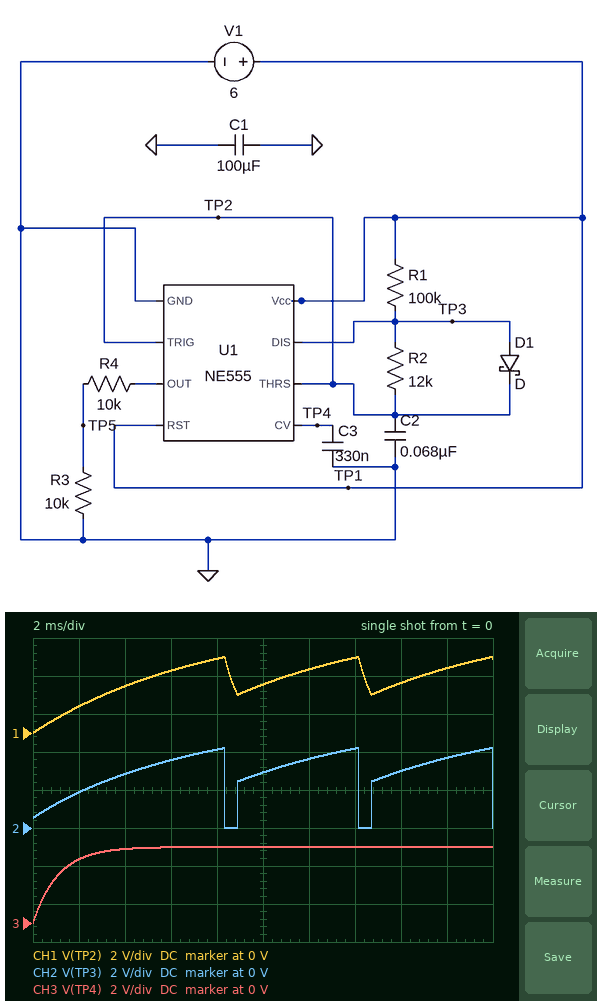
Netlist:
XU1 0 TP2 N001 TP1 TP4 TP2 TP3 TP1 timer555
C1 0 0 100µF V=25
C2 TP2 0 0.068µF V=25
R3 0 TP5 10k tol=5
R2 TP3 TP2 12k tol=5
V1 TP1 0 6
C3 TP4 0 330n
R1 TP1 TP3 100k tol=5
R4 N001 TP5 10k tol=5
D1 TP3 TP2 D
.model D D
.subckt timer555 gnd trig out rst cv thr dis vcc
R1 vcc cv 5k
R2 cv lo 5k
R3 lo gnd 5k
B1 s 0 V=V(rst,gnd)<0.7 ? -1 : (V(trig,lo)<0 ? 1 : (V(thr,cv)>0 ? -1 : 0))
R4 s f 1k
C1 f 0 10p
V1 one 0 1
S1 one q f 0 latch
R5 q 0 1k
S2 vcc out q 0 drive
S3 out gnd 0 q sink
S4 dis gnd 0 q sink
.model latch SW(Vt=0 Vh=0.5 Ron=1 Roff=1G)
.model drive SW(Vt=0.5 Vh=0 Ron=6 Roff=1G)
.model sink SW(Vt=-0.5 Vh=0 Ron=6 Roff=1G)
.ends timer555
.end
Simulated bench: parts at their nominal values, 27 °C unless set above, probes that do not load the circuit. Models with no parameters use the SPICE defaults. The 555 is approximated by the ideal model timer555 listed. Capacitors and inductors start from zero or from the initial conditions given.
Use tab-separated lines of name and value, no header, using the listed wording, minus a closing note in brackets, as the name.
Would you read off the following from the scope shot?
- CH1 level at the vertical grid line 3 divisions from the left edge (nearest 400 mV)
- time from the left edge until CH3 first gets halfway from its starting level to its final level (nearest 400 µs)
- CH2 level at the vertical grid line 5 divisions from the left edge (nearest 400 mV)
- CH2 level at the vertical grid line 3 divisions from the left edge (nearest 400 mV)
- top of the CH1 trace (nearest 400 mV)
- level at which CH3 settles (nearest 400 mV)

CH1 level at the vertical grid line 3 divisions from the left edge	3.2 V
time from the left edge until CH3 first gets halfway from its starting level to its final level	800 µs
CH2 level at the vertical grid line 5 divisions from the left edge	2.8 V
CH2 level at the vertical grid line 3 divisions from the left edge	3.6 V
top of the CH1 trace	4.0 V
level at which CH3 settles	4.0 V
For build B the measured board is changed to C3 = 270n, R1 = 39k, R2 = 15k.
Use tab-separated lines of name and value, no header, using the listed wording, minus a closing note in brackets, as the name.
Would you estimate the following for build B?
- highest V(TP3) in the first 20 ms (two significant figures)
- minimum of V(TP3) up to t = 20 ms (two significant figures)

highest V(TP3) in the first 20 ms	4.5 V
minimum of V(TP3) up to t = 20 ms	1.7 mV
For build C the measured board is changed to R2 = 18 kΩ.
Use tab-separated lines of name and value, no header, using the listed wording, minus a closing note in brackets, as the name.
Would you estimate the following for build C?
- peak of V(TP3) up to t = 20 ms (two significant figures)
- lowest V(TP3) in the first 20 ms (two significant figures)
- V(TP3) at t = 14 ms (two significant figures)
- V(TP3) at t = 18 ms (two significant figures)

peak of V(TP3) up to t = 20 ms	4.3 V
lowest V(TP3) in the first 20 ms	1.0 mV
V(TP3) at t = 14 ms	4.1 V
V(TP3) at t = 18 ms	3.4 V
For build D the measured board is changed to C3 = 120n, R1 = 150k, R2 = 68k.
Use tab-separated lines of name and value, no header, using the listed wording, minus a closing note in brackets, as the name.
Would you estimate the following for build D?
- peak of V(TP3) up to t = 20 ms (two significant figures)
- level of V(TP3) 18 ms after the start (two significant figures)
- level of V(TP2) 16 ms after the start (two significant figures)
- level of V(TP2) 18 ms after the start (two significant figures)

peak of V(TP3) up to t = 20 ms	4.5 V
level of V(TP3) 18 ms after the start	3.0 V
level of V(TP2) 16 ms after the start	2.3 V
level of V(TP2) 18 ms after the start	2.4 V
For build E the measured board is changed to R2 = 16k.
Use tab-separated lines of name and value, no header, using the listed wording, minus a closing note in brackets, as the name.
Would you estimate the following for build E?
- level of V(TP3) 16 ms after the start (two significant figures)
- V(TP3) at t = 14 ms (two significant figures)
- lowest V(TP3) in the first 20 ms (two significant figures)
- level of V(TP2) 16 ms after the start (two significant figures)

level of V(TP3) 16 ms after the start	2.7 V
V(TP3) at t = 14 ms	4.1 V
lowest V(TP3) in the first 20 ms	1.1 mV
level of V(TP2) 16 ms after the start	2.2 V
